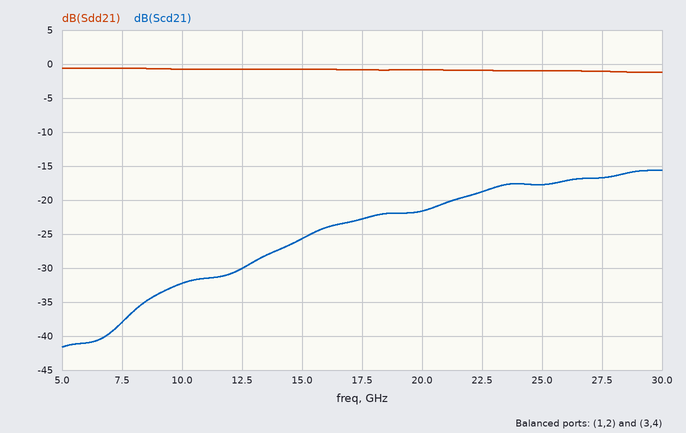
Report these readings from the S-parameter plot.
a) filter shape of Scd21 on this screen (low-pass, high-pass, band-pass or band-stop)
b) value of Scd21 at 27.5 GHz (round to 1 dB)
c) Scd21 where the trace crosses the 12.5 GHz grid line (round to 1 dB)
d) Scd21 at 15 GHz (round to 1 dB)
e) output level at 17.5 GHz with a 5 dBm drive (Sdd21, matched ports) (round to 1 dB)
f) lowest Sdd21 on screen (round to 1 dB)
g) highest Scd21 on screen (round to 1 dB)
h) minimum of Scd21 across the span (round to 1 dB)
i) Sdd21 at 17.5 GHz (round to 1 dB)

high-pass
-17 dB
-30 dB
-26 dB
4 dBm
-1 dB
-16 dB
-42 dB
-1 dB
